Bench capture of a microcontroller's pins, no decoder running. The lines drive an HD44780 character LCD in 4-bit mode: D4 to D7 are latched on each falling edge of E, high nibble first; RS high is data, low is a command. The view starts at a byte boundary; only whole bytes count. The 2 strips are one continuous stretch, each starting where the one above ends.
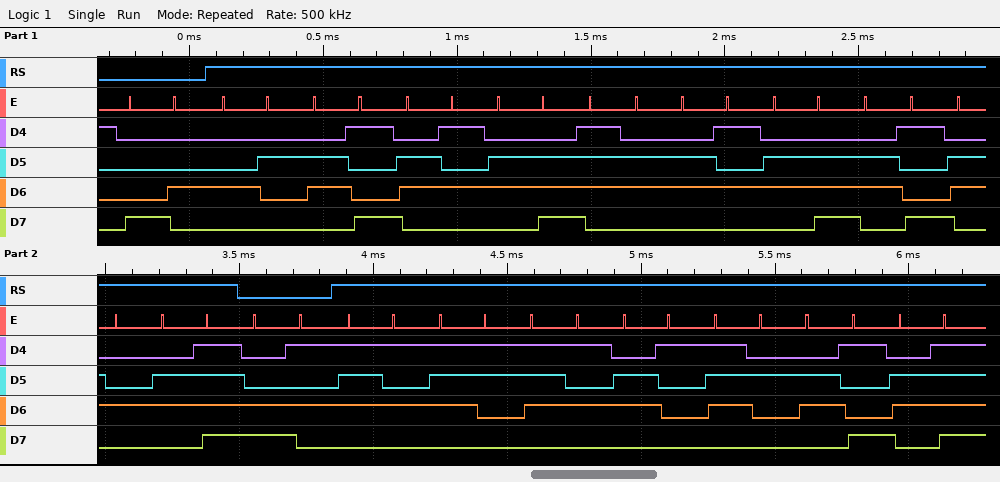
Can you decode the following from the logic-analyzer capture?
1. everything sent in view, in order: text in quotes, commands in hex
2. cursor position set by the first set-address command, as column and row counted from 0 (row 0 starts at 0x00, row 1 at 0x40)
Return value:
0x84 "Bienvenido" 0xC5 "usuario"
column 4, row 0
